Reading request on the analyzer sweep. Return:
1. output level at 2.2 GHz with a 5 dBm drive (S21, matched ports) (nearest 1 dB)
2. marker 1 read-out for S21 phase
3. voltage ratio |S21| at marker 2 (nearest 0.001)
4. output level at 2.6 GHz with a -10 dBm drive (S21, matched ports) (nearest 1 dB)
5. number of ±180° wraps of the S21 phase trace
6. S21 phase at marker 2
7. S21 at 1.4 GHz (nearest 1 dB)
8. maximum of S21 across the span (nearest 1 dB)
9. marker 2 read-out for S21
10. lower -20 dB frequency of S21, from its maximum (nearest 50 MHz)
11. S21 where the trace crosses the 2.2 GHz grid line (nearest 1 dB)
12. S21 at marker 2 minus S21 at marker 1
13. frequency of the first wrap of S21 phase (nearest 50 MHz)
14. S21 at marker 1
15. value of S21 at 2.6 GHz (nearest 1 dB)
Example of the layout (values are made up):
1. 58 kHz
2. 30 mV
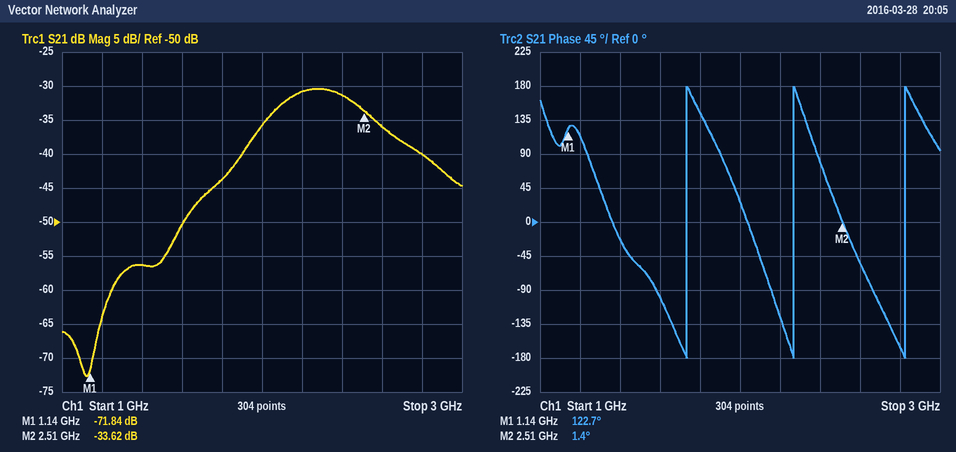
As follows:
1. -26 dBm
2. 122.7°
3. 0.021
4. -46 dBm
5. 3
6. 1.4°
7. -56 dB
8. -30 dB
9. -33.62 dB
10. 1.60 GHz
11. -31 dB
12. 38.22 dB
13. 1.75 GHz
14. -71.84 dB
15. -36 dB
